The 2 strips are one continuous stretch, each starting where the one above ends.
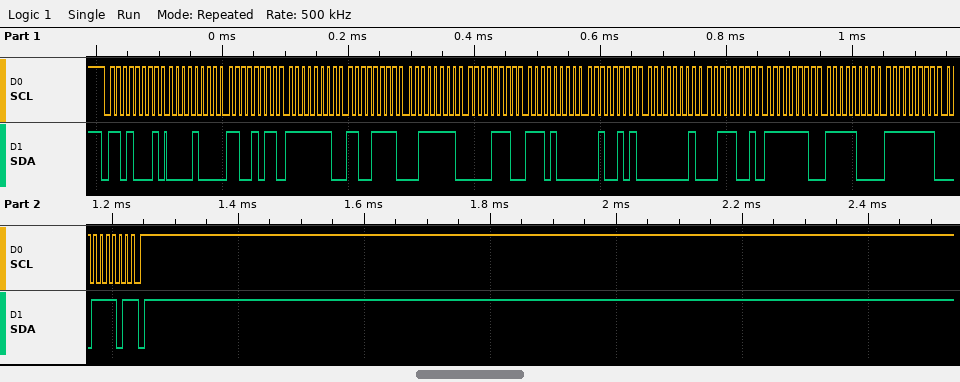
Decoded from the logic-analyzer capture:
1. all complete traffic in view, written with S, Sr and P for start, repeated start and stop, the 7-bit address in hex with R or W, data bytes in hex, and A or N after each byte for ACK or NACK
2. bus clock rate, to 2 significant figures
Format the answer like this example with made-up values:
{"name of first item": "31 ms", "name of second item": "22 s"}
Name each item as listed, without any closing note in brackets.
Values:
{"all complete traffic in view, written with S, Sr and P for start, repeated start and stop, the 7-bit address in hex with R or W, data bytes in hex, and A or N after each byte for ACK or NACK": "S 68R A 08 A CB A FE A CF A 3F A 0E A E8 A 25 A 01 A 39 A FE A F8 A FF A 3D N P", "bus clock rate, to 2 significant figures": "100 kHz"}
